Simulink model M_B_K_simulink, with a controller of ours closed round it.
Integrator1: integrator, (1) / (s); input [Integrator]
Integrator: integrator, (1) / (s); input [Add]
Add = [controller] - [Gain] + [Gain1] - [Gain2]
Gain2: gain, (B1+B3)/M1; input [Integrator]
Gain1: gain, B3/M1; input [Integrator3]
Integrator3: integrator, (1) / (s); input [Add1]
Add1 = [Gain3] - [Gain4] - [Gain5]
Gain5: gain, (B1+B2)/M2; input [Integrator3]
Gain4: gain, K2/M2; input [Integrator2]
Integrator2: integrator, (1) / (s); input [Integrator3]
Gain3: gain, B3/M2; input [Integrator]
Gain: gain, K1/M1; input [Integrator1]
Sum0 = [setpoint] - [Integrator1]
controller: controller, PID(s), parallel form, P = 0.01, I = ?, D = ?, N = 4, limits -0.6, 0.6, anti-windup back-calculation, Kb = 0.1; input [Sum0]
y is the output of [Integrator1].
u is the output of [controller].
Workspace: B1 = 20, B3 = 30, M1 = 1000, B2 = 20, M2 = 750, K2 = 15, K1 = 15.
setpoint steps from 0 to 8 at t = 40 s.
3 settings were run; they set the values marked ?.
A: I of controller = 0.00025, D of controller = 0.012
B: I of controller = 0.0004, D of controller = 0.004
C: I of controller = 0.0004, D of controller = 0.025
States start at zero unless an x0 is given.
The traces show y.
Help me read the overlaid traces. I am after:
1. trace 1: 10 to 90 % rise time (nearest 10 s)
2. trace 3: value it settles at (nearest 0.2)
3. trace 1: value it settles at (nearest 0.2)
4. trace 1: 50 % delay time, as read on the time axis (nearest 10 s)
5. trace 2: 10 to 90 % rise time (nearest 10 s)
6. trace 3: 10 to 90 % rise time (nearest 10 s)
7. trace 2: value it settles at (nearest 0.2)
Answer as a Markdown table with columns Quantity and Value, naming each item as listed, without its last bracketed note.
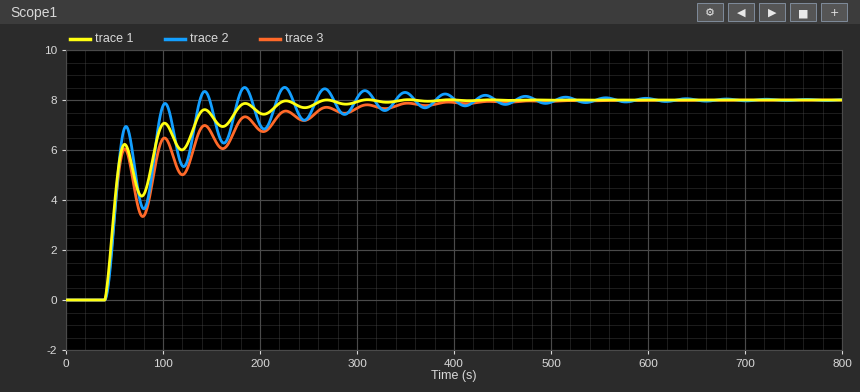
| Quantity | Value |
|---|---|
| trace 1: 10 to 90 % rise time | 90 s |
| trace 3: value it settles at | 8.0 |
| trace 1: value it settles at | 8.0 |
| trace 1: 50 % delay time, as read on the time axis | 50 s |
| trace 2: 10 to 90 % rise time | 50 s |
| trace 3: 10 to 90 % rise time | 140 s |
| trace 2: value it settles at | 8.0 |
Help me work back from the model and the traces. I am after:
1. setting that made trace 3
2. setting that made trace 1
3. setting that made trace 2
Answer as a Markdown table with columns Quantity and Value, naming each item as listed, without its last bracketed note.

| Quantity | Value |
|---|---|
| setting that made trace 3 | A |
| setting that made trace 1 | C |
| setting that made trace 2 | B |
